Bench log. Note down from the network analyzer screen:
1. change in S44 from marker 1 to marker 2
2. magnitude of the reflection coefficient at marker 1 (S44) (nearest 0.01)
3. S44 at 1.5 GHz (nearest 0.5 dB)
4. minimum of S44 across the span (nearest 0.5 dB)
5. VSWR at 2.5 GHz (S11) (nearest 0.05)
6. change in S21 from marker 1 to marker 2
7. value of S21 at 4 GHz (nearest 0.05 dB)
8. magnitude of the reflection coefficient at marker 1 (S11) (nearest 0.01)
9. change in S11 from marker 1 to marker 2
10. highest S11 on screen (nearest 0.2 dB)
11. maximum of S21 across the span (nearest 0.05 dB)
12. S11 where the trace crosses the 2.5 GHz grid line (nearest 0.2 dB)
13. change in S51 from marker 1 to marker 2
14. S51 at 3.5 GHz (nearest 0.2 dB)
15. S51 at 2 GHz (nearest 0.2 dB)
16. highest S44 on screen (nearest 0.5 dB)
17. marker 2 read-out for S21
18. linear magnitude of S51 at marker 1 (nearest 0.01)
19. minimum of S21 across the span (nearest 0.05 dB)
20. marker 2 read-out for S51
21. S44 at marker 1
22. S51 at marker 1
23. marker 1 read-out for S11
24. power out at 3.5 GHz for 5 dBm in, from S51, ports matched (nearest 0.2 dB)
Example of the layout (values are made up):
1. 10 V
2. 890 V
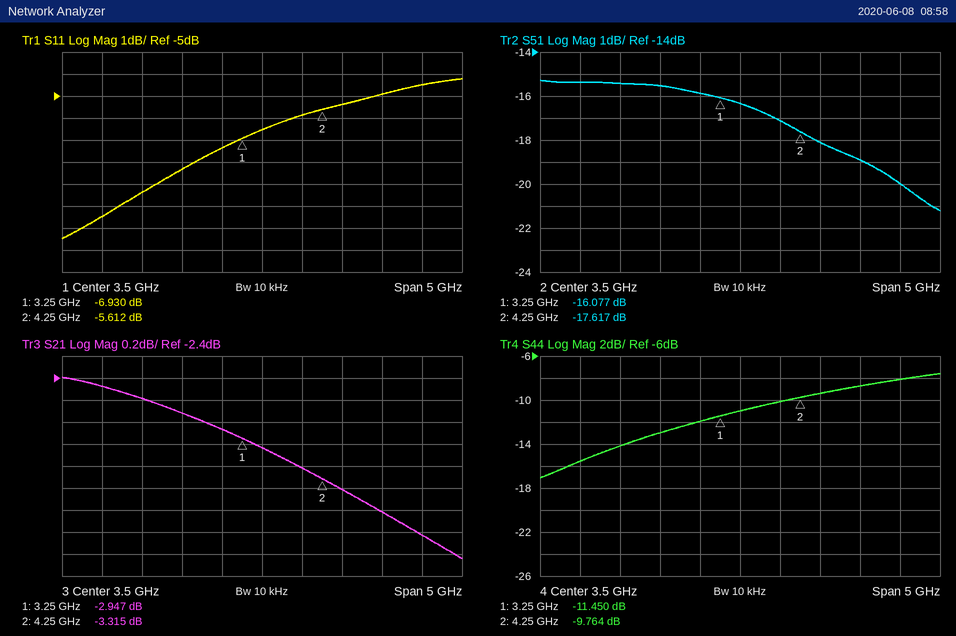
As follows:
1. 1.686 dB
2. 0.27
3. -15.5 dB
4. -17.0 dB
5. 2.25
6. -0.368 dB
7. -3.20 dB
8. 0.45
9. 1.318 dB
10. -4.2 dB
11. -2.40 dB
12. -8.4 dB
13. -1.540 dB
14. -16.4 dB
15. -15.4 dB
16. -7.5 dB
17. -3.315 dB
18. 0.16
19. -4.05 dB
20. -17.617 dB
21. -11.450 dB
22. -16.077 dB
23. -6.930 dB
24. -11.4 dBm
